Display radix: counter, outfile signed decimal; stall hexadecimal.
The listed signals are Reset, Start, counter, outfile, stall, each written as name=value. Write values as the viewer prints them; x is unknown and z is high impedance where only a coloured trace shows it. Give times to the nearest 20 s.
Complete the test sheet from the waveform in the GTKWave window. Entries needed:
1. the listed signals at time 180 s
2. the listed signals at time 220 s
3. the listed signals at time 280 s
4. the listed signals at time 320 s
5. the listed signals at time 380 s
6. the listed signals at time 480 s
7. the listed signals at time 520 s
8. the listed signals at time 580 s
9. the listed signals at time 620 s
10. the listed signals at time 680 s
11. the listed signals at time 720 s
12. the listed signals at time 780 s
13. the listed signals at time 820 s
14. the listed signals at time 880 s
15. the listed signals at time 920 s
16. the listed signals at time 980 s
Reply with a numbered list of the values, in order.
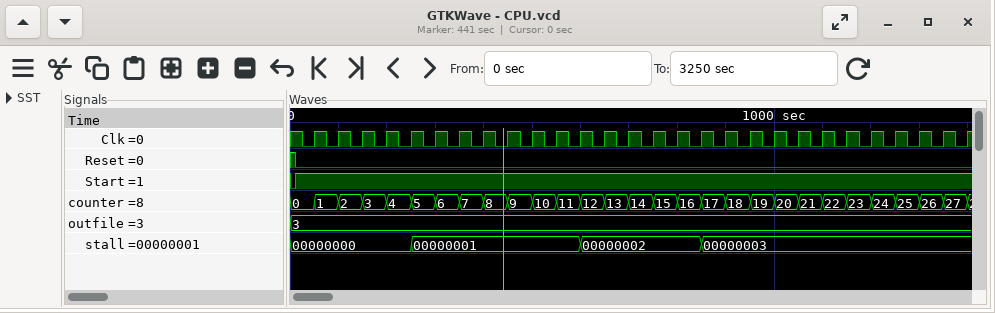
1. Reset=0, Start=1, counter=3, outfile=3, stall=00000000
2. Reset=0, Start=1, counter=4, outfile=3, stall=00000000
3. Reset=0, Start=1, counter=5, outfile=3, stall=00000001
4. Reset=0, Start=1, counter=6, outfile=3, stall=00000001
5. Reset=0, Start=1, counter=7, outfile=3, stall=00000001
6. Reset=0, Start=1, counter=9, outfile=3, stall=00000001
7. Reset=0, Start=1, counter=10, outfile=3, stall=00000001
8. Reset=0, Start=1, counter=11, outfile=3, stall=00000001
9. Reset=0, Start=1, counter=12, outfile=3, stall=00000002
10. Reset=0, Start=1, counter=13, outfile=3, stall=00000002
11. Reset=0, Start=1, counter=14, outfile=3, stall=00000002
12. Reset=0, Start=1, counter=15, outfile=3, stall=00000002
13. Reset=0, Start=1, counter=16, outfile=3, stall=00000002
14. Reset=0, Start=1, counter=17, outfile=3, stall=00000003
15. Reset=0, Start=1, counter=18, outfile=3, stall=00000003
16. Reset=0, Start=1, counter=19, outfile=3, stall=00000003
